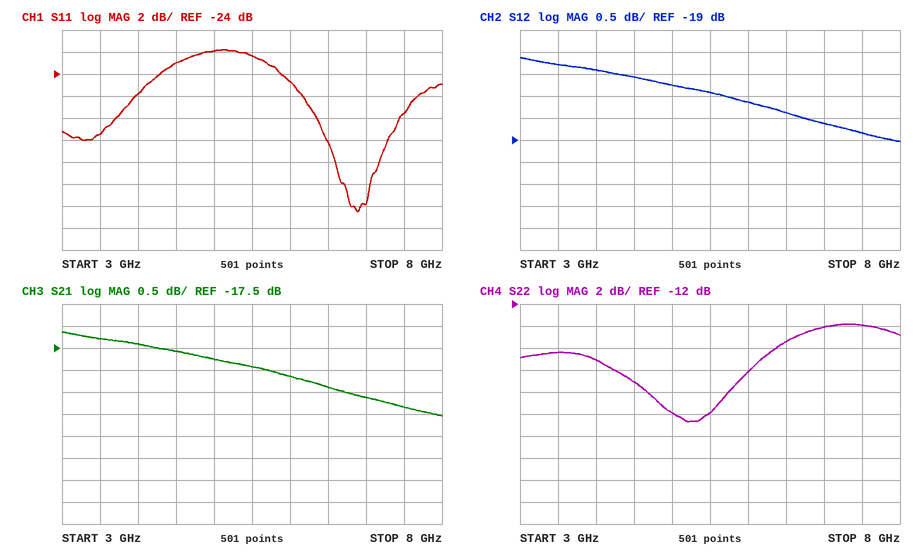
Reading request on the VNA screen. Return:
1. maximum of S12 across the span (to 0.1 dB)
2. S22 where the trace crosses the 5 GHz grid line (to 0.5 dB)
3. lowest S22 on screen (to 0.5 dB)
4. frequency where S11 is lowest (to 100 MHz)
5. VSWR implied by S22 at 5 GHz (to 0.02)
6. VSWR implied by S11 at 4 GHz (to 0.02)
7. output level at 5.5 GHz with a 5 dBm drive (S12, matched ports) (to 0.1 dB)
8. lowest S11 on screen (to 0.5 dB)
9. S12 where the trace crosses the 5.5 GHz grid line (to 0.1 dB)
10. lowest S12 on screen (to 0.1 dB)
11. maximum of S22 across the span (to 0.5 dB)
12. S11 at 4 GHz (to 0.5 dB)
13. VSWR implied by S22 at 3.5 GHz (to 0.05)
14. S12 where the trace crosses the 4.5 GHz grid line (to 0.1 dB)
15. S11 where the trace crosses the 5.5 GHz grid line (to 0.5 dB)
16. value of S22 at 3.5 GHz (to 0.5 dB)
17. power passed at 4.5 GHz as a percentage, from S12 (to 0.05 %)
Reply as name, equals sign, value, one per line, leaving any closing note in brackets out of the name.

maximum of S12 across the span = -17.1 dB
S22 where the trace crosses the 5 GHz grid line = -22.0 dB
lowest S22 on screen = -22.5 dB
frequency where S11 is lowest = 6.9 GHz
VSWR implied by S22 at 5 GHz = 1.18
VSWR implied by S11 at 4 GHz = 1.10
output level at 5.5 GHz with a 5 dBm drive (S12, matched ports) = -12.9 dBm
lowest S11 on screen = -36.5 dB
S12 where the trace crosses the 5.5 GHz grid line = -17.9 dB
lowest S12 on screen = -19.0 dB
maximum of S22 across the span = -14.0 dB
S11 at 4 GHz = -26.0 dB
VSWR implied by S22 at 3.5 GHz = 1.35
S12 where the trace crosses the 4.5 GHz grid line = -17.6 dB
S11 where the trace crosses the 5.5 GHz grid line = -22.5 dB
value of S22 at 3.5 GHz = -16.5 dB
power passed at 4.5 GHz as a percentage, from S12 = 1.75 %
